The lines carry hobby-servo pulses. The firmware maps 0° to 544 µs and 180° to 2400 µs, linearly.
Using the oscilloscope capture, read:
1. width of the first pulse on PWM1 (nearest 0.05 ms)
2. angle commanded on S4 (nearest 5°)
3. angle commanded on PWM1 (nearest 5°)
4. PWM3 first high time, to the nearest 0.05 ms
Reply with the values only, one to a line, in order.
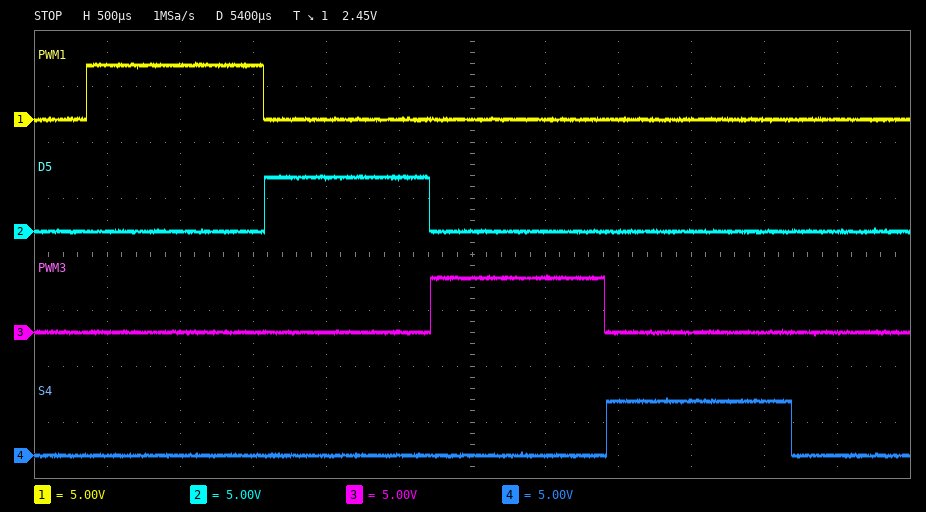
1.20 ms
70°
65°
1.20 ms
